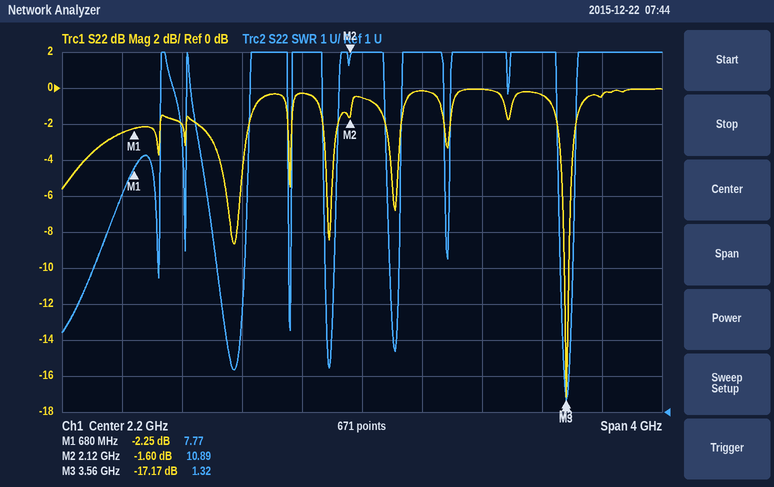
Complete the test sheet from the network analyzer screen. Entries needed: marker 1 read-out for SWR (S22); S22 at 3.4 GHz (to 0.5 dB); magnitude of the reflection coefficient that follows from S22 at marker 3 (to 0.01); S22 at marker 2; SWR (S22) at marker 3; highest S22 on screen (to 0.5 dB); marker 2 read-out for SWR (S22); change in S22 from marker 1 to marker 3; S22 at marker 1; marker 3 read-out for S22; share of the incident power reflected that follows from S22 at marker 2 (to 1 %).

7.77
-0.5 dB
0.14
-1.60 dB
1.32
0.0 dB
10.89
-14.92 dB
-2.25 dB
-17.17 dB
69 %
